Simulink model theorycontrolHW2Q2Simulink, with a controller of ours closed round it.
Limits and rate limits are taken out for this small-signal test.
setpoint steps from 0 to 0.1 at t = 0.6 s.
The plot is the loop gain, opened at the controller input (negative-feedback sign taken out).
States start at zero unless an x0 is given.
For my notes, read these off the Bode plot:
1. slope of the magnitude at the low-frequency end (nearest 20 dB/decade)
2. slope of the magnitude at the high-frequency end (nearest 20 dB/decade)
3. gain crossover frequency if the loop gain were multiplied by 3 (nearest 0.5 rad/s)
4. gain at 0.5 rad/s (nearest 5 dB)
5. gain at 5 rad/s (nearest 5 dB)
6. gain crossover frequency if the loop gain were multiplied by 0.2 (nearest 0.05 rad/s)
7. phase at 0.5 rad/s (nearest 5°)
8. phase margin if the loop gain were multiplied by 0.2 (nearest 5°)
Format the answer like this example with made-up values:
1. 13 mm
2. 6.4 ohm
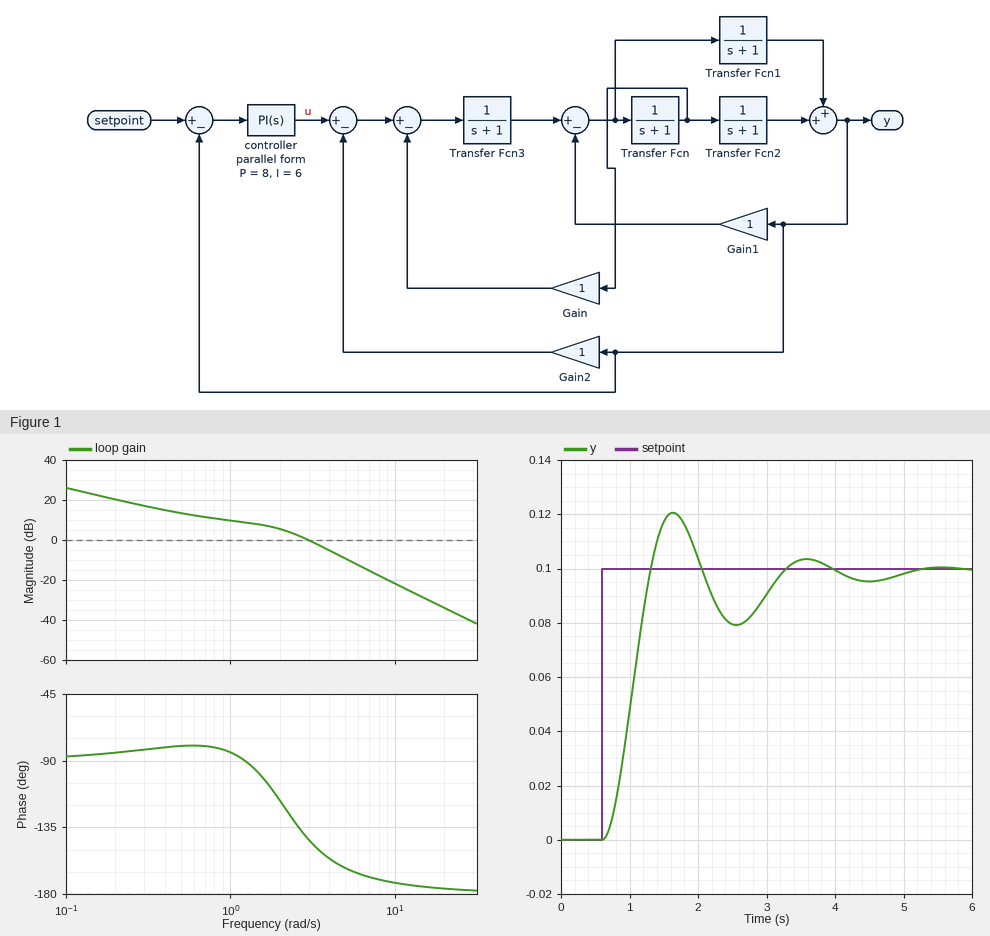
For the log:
1. -20 dB/decade
2. -40 dB/decade
3. 5.0 rad/s
4. 15 dB
5. -10 dB
6. 0.45 rad/s
7. -80°
8. 100°
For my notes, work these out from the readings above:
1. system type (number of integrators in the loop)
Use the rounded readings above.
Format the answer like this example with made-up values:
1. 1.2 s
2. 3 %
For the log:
1. 1
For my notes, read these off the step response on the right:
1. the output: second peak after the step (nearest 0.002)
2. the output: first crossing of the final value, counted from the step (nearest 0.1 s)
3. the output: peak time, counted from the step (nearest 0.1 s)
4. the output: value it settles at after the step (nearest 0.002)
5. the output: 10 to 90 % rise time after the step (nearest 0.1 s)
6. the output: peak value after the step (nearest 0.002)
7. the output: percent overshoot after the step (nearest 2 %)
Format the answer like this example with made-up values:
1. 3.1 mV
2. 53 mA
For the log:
1. 0.104
2. 0.7 s
3. 1.0 s
4. 0.100
5. 0.5 s
6. 0.120
7. 20 %
